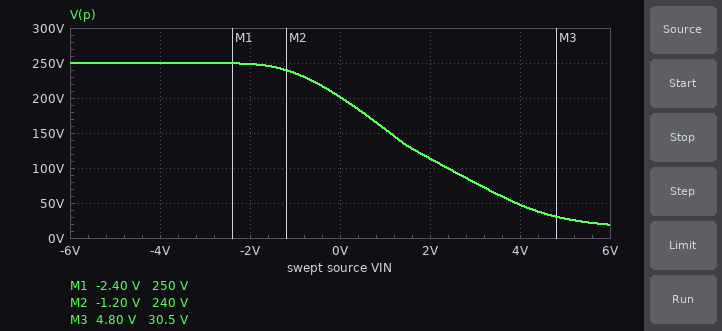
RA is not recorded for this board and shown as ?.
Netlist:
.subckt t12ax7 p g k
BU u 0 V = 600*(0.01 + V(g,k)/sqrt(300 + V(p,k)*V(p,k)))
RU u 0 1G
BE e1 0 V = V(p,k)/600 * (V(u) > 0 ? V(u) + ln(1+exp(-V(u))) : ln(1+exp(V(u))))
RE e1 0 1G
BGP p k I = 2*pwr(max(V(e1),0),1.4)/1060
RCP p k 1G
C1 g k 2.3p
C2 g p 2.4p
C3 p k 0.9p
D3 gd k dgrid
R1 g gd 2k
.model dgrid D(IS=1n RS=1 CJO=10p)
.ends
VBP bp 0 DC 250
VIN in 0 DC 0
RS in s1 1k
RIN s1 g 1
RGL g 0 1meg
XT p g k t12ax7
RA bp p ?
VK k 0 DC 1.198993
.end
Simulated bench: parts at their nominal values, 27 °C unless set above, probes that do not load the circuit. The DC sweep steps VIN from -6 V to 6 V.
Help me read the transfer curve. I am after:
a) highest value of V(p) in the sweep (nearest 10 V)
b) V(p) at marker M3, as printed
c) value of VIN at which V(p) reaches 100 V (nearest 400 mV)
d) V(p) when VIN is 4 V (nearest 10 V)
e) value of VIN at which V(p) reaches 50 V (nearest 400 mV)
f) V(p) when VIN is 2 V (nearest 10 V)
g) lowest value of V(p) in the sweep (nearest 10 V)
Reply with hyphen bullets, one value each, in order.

- 250 V
- 30.5 V
- 2.4 V
- 50 V
- 4.0 V
- 110 V
- 20 V
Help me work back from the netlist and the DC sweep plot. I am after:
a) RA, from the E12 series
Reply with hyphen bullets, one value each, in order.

- 33 kΩ
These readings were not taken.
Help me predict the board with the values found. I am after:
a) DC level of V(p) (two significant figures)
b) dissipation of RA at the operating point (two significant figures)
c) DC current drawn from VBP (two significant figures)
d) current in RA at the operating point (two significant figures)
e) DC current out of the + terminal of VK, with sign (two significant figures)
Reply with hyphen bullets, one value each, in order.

- 200 V
- 71 mW
- 1.5 mA
- 1.5 mA
- -1.5 mA
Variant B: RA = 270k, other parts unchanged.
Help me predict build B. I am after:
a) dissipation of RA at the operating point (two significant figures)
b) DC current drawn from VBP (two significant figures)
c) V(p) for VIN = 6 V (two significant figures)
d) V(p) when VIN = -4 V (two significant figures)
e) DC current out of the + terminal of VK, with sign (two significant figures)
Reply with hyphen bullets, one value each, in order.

- 41 mW
- 390 µA
- 4.2 V
- 250 V
- -390 µA
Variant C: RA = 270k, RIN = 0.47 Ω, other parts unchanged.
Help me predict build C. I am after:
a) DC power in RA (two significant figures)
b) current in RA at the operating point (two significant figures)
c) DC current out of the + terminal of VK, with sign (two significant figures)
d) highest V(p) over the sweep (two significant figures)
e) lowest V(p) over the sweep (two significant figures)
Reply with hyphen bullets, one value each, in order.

- 41 mW
- 390 µA
- -390 µA
- 250 V
- 4.2 V
